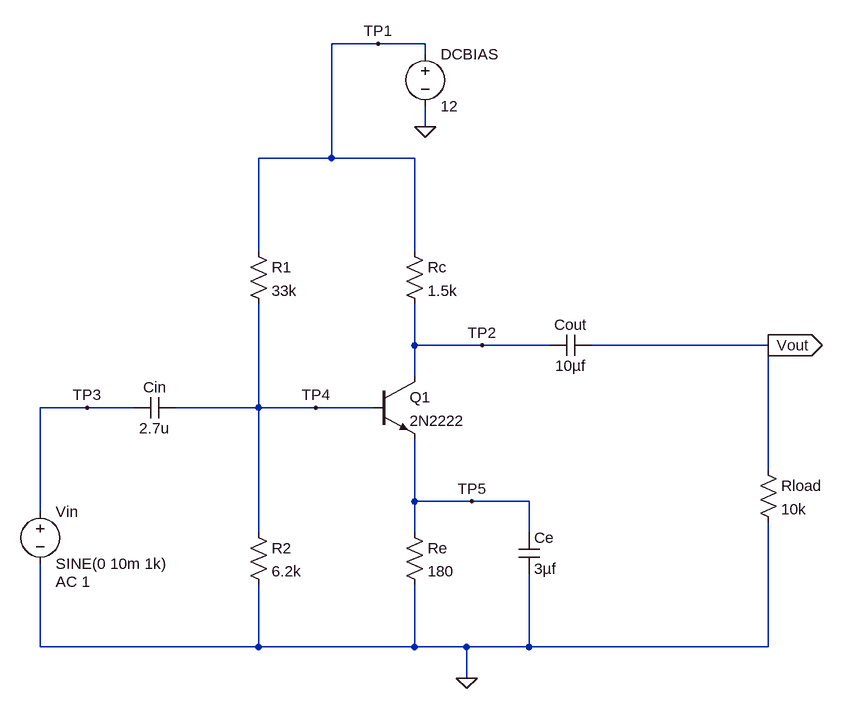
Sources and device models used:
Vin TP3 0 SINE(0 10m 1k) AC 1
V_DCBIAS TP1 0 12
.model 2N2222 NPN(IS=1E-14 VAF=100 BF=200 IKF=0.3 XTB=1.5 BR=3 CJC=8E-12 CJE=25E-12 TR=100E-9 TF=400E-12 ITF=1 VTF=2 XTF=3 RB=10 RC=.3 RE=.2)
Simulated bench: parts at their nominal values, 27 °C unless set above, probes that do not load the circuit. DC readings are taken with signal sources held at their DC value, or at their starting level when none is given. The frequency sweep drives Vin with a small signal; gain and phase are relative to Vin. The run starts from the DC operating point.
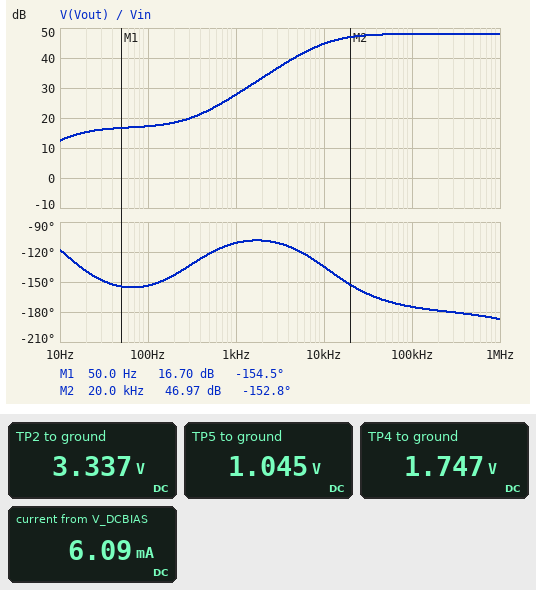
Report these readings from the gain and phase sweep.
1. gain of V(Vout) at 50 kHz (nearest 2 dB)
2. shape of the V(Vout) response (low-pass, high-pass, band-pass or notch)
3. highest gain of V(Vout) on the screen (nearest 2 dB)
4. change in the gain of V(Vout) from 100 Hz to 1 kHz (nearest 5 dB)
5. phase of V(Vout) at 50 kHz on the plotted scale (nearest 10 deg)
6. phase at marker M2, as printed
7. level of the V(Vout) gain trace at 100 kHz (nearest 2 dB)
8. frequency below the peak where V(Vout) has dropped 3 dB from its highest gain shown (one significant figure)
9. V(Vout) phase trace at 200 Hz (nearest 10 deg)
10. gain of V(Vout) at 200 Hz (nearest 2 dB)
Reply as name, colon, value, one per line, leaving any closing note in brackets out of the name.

gain of V(Vout) at 50 kHz: 48 dB
shape of the V(Vout) response: high-pass
highest gain of V(Vout) on the screen: 48 dB
change in the gain of V(Vout) from 100 Hz to 1 kHz: 10 dB
phase of V(Vout) at 50 kHz on the plotted scale: -170 deg
phase at marker M2, as printed: -152.8 deg
level of the V(Vout) gain trace at 100 kHz: 48 dB
frequency below the peak where V(Vout) has dropped 3 dB from its highest gain shown: 10 kHz
V(Vout) phase trace at 200 Hz: -140 deg
gain of V(Vout) at 200 Hz: 18 dB
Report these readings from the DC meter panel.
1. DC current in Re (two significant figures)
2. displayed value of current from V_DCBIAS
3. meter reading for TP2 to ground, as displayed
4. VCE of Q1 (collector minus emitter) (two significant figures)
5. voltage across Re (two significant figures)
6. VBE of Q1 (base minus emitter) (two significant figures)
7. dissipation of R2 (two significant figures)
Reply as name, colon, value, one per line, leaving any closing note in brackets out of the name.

DC current in Re: 5.8 mA
displayed value of current from V_DCBIAS: 6.09 mA
meter reading for TP2 to ground, as displayed: 3.337 V
VCE of Q1 (collector minus emitter): 2.3 V
voltage across Re: 1.0 V
VBE of Q1 (base minus emitter): 700 mV
dissipation of R2: 490 µW
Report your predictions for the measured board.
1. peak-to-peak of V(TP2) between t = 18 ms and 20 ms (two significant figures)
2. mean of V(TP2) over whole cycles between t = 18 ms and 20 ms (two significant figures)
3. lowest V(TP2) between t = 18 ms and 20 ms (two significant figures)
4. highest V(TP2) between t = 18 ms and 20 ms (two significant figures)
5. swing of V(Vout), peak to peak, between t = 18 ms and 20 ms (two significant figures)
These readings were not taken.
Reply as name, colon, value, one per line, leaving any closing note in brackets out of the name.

peak-to-peak of V(TP2) between t = 18 ms and 20 ms: 490 mV
mean of V(TP2) over whole cycles between t = 18 ms and 20 ms: 3.3 V
lowest V(TP2) between t = 18 ms and 20 ms: 3.1 V
highest V(TP2) between t = 18 ms and 20 ms: 3.6 V
swing of V(Vout), peak to peak, between t = 18 ms and 20 ms: 490 mV
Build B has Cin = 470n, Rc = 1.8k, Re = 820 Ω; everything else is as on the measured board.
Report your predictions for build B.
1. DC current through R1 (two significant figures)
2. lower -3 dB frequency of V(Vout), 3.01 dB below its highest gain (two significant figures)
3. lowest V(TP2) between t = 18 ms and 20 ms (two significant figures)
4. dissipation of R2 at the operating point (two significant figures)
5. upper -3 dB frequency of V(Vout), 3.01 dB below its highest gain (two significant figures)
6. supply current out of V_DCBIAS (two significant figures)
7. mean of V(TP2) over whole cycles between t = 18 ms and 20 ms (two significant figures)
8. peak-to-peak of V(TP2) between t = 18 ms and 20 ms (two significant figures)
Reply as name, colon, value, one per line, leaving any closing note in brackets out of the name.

DC current through R1: 310 µA
lower -3 dB frequency of V(Vout), 3.01 dB below its highest gain: 3.0 kHz
lowest V(TP2) between t = 18 ms and 20 ms: 9.1 V
dissipation of R2 at the operating point: 560 µW
upper -3 dB frequency of V(Vout), 3.01 dB below its highest gain: 18 MHz
supply current out of V_DCBIAS: 1.8 mA
mean of V(TP2) over whole cycles between t = 18 ms and 20 ms: 9.4 V
peak-to-peak of V(TP2) between t = 18 ms and 20 ms: 520 mV
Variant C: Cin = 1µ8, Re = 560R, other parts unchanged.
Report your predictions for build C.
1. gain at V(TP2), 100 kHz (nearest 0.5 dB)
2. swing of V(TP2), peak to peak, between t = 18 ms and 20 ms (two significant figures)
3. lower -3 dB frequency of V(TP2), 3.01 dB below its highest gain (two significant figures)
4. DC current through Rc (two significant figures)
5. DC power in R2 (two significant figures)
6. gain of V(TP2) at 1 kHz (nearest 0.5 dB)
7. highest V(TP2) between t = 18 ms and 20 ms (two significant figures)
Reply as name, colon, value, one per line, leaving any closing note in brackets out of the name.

gain at V(TP2), 100 kHz: 40.0 dB
swing of V(TP2), peak to peak, between t = 18 ms and 20 ms: 460 mV
lower -3 dB frequency of V(TP2), 3.01 dB below its highest gain: 4.2 kHz
DC current through Rc: 2.1 mA
DC power in R2: 550 µW
gain of V(TP2) at 1 kHz: 27.5 dB
highest V(TP2) between t = 18 ms and 20 ms: 9.1 V
